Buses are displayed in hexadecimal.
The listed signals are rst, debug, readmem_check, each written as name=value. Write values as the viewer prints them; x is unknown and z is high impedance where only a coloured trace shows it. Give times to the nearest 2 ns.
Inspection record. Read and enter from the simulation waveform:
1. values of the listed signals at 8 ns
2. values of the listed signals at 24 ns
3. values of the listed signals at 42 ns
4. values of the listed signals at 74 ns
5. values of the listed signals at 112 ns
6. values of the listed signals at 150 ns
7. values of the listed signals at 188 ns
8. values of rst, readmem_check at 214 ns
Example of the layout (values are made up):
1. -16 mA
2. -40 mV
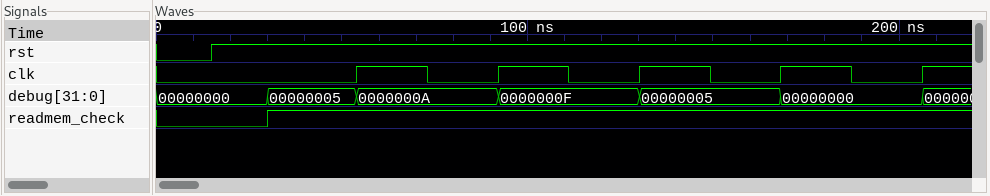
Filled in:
1. rst=0, debug=00000000, readmem_check=0
2. rst=1, debug=00000000, readmem_check=0
3. rst=1, debug=00000005, readmem_check=1
4. rst=1, debug=0000000A, readmem_check=1
5. rst=1, debug=0000000F, readmem_check=1
6. rst=1, debug=00000005, readmem_check=1
7. rst=1, debug=00000000, readmem_check=1
8. rst=1, readmem_check=1
